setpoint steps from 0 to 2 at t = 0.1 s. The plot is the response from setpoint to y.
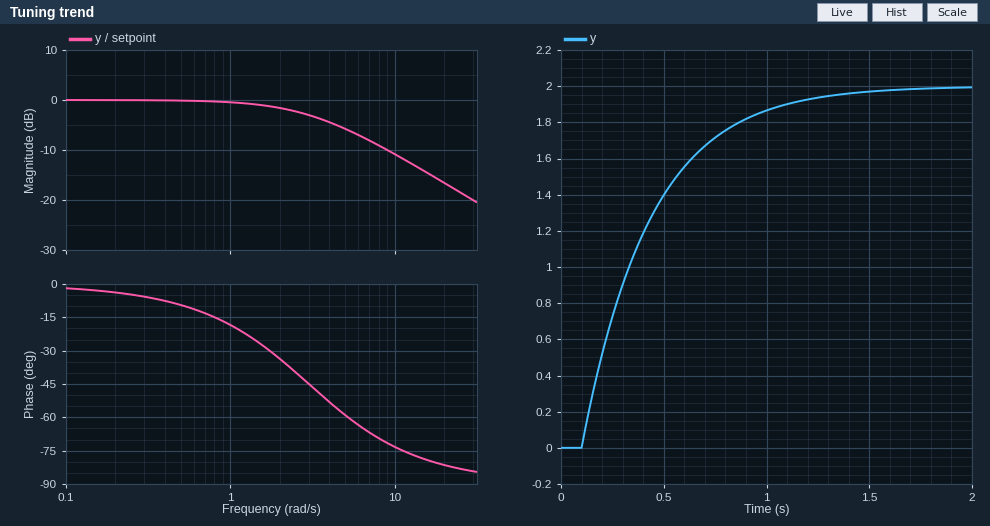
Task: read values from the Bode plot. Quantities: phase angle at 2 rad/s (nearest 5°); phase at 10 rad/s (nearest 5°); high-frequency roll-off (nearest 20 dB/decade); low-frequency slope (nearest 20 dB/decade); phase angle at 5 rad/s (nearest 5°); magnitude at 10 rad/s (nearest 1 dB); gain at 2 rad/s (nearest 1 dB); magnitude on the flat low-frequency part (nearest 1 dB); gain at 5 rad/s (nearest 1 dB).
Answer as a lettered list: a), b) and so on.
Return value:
a) -35°
b) -75°
c) -20 dB/decade
d) 0 dB/decade
e) -60°
f) -11 dB
g) -2 dB
h) 0 dB
i) -6 dB
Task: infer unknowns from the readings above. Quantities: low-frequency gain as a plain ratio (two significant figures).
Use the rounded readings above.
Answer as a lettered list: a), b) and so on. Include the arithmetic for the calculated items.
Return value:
a) 10^(0 / 20) = 1.0
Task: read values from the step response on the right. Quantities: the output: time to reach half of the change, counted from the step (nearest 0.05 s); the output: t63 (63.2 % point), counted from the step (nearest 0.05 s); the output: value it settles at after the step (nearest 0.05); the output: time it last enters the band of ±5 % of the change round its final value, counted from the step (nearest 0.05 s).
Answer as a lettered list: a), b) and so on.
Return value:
a) 0.25 s
b) 0.35 s
c) 2.00
d) 1.00 s
